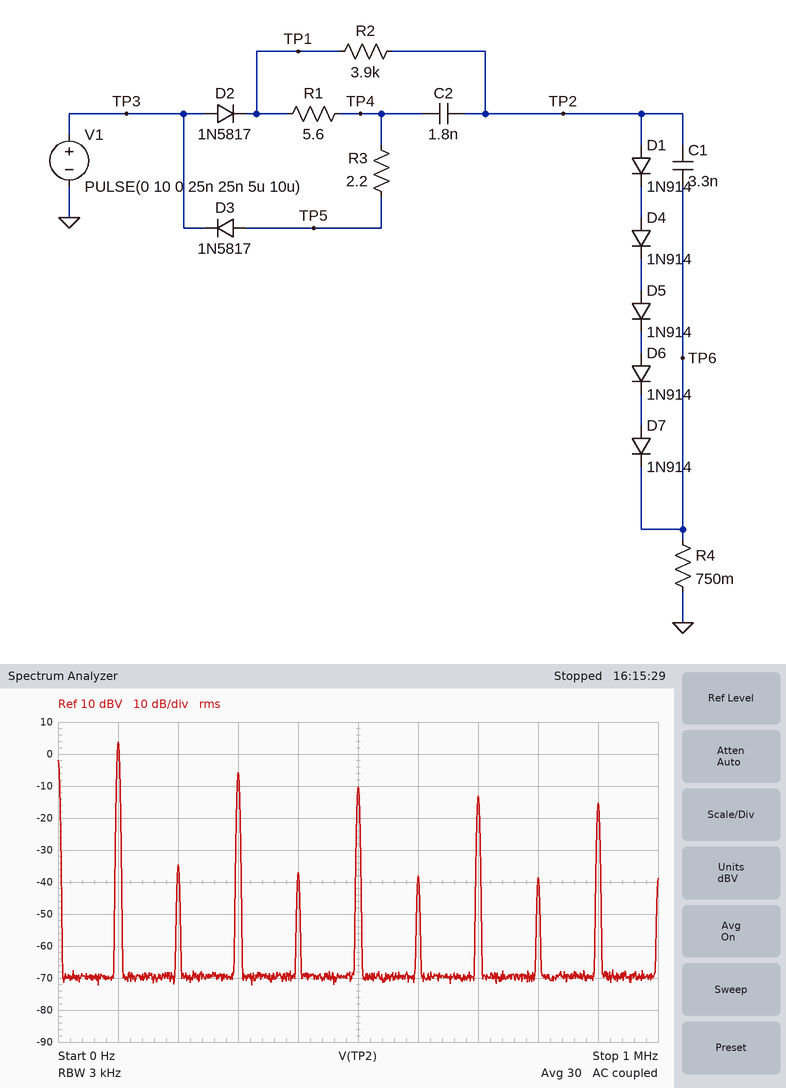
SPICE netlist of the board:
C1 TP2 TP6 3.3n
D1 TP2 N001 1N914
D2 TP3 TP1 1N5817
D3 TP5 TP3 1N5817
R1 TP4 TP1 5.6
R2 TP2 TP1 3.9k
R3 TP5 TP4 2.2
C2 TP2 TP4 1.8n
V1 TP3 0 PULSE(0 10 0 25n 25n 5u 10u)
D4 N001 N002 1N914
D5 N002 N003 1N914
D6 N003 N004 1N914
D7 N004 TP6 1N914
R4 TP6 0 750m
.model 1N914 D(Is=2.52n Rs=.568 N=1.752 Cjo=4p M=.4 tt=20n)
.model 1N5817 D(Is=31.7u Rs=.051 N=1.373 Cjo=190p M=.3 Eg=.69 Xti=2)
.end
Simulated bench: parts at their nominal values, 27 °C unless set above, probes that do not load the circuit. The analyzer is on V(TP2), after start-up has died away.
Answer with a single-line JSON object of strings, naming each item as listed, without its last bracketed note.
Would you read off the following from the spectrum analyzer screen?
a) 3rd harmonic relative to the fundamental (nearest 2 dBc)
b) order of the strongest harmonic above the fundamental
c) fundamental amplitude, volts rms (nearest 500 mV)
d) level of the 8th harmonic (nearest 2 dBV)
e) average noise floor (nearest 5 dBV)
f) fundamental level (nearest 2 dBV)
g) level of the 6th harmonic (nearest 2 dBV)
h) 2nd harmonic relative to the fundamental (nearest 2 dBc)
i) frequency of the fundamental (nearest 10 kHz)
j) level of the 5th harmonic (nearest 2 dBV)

{"3rd harmonic relative to the fundamental": "-10 dBc", "order of the strongest harmonic above the fundamental": "3", "fundamental amplitude, volts rms": "1.5 V", "level of the 8th harmonic": "-38 dBV", "average noise floor": "-70 dBV", "fundamental level": "4 dBV", "level of the 6th harmonic": "-38 dBV", "2nd harmonic relative to the fundamental": "-38 dBc", "frequency of the fundamental": "100 kHz", "level of the 5th harmonic": "-10 dBV"}
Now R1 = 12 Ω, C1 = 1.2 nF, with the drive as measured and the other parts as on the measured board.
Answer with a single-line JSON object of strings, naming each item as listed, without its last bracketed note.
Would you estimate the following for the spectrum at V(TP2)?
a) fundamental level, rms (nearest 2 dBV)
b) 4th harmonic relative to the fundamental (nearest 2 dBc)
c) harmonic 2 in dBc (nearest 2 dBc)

{"fundamental level, rms": "8 dBV", "4th harmonic relative to the fundamental": "-34 dBc", "harmonic 2 in dBc": "-28 dBc"}
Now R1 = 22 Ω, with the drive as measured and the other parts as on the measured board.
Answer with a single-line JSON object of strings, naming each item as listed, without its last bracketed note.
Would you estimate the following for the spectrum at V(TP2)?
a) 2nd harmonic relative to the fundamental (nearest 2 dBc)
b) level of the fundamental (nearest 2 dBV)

{"2nd harmonic relative to the fundamental": "-44 dBc", "level of the fundamental": "4 dBV"}
